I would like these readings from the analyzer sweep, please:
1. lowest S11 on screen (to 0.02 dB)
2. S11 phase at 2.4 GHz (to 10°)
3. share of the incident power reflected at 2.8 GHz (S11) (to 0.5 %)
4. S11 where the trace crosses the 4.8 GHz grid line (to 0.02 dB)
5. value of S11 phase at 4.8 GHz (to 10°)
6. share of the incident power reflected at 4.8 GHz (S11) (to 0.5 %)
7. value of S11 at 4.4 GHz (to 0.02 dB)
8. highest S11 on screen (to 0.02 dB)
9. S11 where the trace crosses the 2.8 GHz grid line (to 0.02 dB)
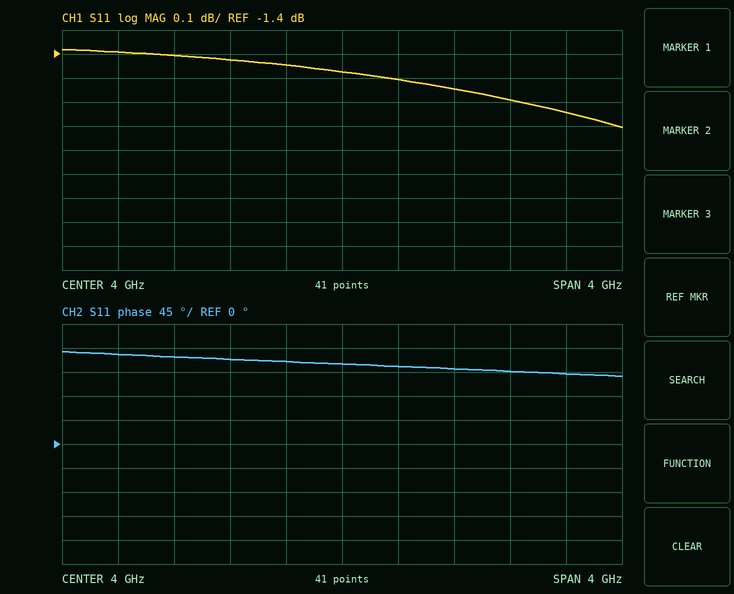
-1.70 dB
170°
72.5 %
-1.54 dB
140°
70.0 %
-1.50 dB
-1.38 dB
-1.40 dB
